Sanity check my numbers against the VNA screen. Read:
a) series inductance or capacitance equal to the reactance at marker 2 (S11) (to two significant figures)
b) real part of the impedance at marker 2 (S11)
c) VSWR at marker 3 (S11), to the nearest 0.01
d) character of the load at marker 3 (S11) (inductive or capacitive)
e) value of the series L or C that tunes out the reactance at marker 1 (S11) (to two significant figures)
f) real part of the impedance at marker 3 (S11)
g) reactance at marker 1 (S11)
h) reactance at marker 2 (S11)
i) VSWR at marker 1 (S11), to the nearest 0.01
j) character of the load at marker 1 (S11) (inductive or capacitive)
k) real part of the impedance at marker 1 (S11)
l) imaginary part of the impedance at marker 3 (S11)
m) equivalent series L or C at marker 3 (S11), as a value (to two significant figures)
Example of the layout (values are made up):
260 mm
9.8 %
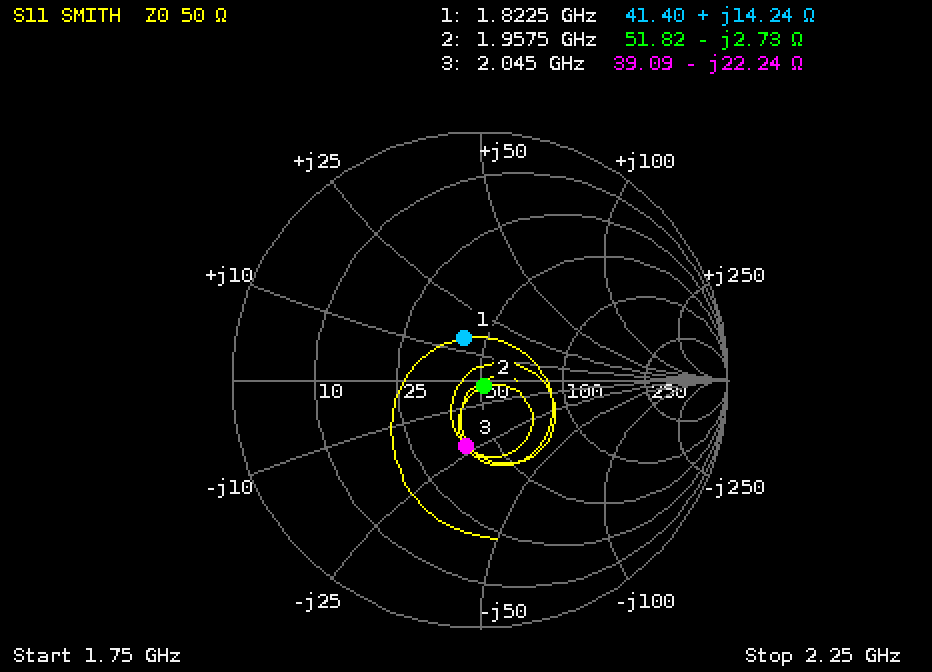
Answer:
30 pF
51.82 Ω
1.74
capacitive
6.1 pF
39.09 Ω
+14.24 Ω
-2.73 Ω
1.44
inductive
41.40 Ω
-22.24 Ω
3.5 pF
